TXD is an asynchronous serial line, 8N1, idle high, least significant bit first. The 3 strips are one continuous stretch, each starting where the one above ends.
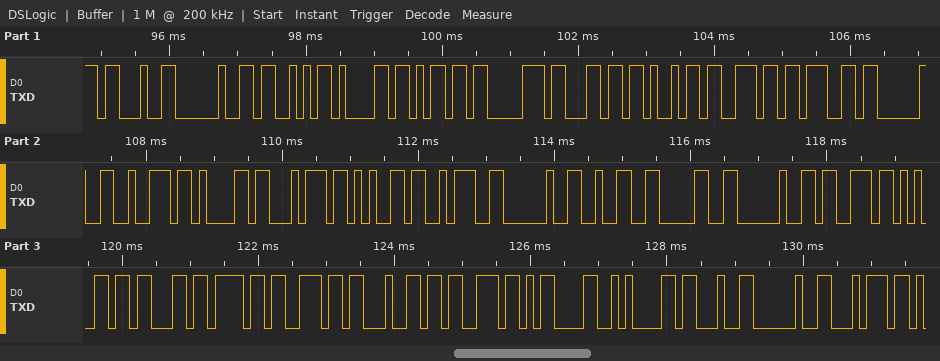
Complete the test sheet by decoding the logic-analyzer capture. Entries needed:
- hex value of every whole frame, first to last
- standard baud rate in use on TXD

23 20 53 61 6D 70 6C 69 6E 67 20 72 61 74 65 3A 20 32 30 20 73 65 63 6F 6E 64 73 0D 0A 23 20 74
9600 baud
